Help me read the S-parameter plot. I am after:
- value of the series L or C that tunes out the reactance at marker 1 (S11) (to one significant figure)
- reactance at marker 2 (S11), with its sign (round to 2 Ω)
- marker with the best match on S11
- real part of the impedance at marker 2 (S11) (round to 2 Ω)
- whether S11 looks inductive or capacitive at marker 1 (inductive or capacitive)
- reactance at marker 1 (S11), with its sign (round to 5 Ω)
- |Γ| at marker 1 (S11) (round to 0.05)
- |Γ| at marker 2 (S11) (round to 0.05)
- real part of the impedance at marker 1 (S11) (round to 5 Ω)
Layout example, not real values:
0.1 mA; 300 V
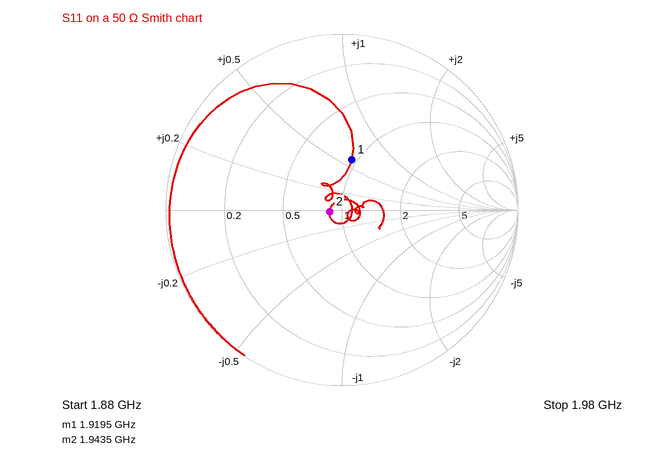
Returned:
3 pF; 0 Ω; marker 2; 44 Ω; inductive; +30 Ω; 0.30; 0.05; 45 Ω
